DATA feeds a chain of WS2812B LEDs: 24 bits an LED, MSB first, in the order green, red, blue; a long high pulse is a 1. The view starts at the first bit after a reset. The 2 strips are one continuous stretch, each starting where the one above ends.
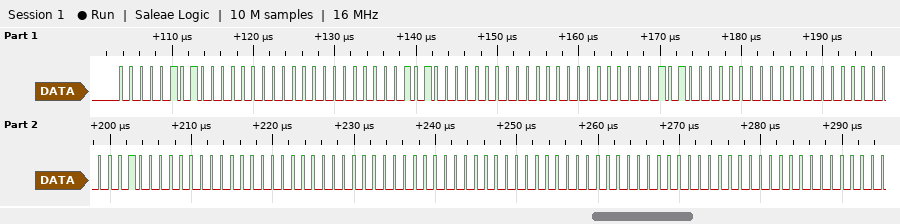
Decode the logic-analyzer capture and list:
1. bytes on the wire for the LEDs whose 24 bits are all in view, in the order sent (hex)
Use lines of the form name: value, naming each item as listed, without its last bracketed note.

bytes on the wire for the LEDs whose 24 bits are all in view, in the order sent: 05 00 00 0A 00 00 05 00 00 01 00 00 00 00 00 00 00 00
